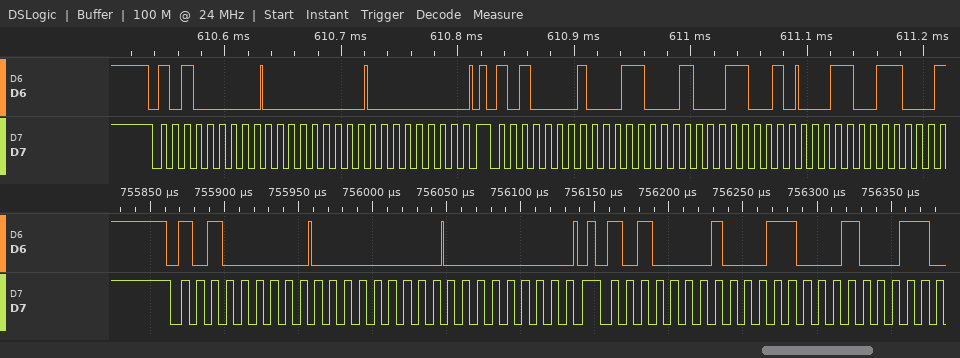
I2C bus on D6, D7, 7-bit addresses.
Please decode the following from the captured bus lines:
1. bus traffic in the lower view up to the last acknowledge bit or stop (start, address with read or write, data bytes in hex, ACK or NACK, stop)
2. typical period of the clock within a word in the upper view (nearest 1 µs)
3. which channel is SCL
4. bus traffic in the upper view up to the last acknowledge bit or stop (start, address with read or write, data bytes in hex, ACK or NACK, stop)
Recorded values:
start, address 50 write ACK, 00 ACK, 00 ACK, stop, start, address 50 read ACK, 31 ACK
10 µs
D7
start, address 50 write ACK, 00 ACK, 00 ACK, stop, start, address 50 read ACK, 31 ACK, 32 ACK, 33 ACK
